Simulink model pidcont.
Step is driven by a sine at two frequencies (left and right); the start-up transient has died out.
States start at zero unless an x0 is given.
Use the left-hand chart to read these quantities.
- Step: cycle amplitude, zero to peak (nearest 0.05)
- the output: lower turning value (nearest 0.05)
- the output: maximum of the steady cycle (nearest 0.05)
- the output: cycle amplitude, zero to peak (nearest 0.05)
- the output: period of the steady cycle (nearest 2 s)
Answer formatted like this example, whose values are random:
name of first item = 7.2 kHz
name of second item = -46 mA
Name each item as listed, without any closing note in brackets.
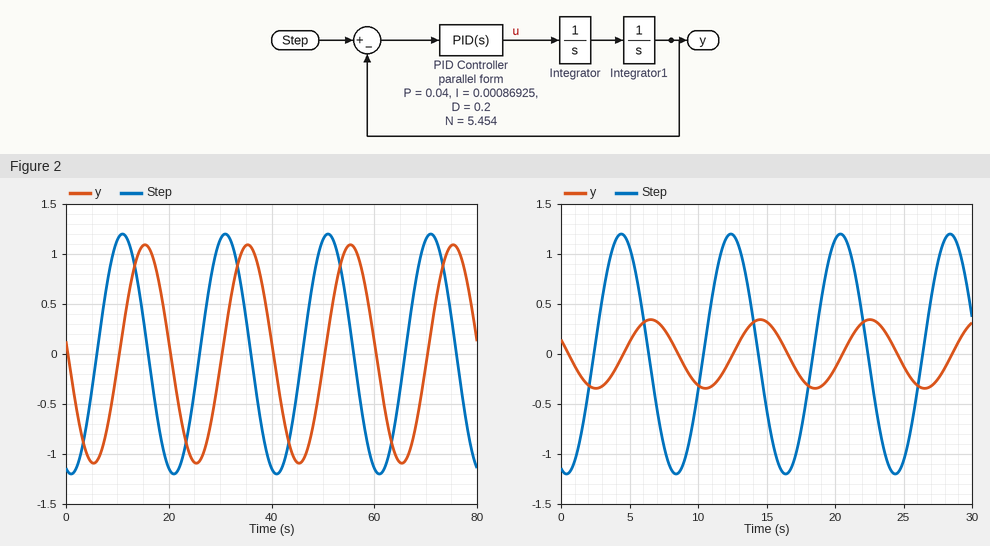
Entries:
Step: cycle amplitude, zero to peak = 1.20
the output: lower turning value = -1.10
the output: maximum of the steady cycle = 1.10
the output: cycle amplitude, zero to peak = 1.10
the output: period of the steady cycle = 20 s
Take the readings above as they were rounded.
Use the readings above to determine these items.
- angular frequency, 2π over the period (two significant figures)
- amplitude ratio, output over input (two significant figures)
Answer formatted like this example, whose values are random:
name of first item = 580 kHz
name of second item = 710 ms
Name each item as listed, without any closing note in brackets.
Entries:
angular frequency, 2π over the period = 0.31 rad/s
amplitude ratio, output over input = 0.92
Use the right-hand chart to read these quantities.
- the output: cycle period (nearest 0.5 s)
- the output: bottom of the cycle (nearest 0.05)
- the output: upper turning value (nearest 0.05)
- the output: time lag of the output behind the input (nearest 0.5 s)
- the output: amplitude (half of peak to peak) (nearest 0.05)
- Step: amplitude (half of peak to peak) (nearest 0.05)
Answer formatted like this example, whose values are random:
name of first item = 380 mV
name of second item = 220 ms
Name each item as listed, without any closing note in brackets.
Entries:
the output: cycle period = 8.0 s
the output: bottom of the cycle = -0.35
the output: upper turning value = 0.35
the output: time lag of the output behind the input = 2.0 s
the output: amplitude (half of peak to peak) = 0.35
Step: amplitude (half of peak to peak) = 1.20
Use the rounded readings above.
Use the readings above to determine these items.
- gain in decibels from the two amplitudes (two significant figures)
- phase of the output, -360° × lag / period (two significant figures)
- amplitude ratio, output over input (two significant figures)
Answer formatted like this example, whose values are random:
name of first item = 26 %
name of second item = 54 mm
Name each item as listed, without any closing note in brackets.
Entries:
gain in decibels from the two amplitudes = -11 dB
phase of the output, -360° × lag / period = -90°
amplitude ratio, output over input = 0.29
